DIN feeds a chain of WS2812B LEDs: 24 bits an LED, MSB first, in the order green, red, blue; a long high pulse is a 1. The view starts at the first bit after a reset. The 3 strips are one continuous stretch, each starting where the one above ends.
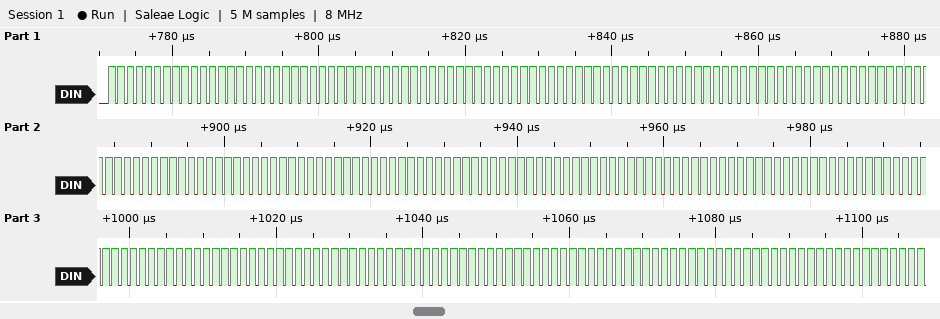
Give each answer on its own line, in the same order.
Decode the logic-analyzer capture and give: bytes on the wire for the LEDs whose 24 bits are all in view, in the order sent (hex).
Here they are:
FF FF FF FF FF FF FF FF FF FF FF FF FF FF FF FF FF FF FF FF FF FF FF FF FF FF FF FF FF FF FF FF FF
